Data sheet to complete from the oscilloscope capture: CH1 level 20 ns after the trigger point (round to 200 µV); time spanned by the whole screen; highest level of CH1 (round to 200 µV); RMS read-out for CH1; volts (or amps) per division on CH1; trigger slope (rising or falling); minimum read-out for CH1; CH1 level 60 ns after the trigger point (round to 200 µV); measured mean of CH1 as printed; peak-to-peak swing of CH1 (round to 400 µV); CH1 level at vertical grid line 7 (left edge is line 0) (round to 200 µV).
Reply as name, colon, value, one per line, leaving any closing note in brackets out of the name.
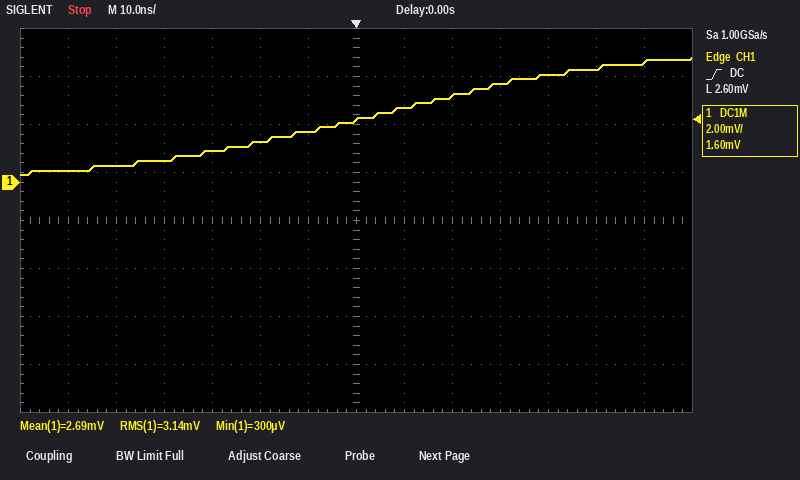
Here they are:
CH1 level 20 ns after the trigger point: 3.6 mV
time spanned by the whole screen: 140 ns
highest level of CH1: 5.2 mV
RMS read-out for CH1: 3.14 mV
volts (or amps) per division on CH1: 2 mV
trigger slope: rising
minimum read-out for CH1: 300 µV
CH1 level 60 ns after the trigger point: 5.0 mV
measured mean of CH1 as printed: 2.69 mV
peak-to-peak swing of CH1: 4.8 mV
CH1 level at vertical grid line 7 (left edge is line 0): 2.6 mV
